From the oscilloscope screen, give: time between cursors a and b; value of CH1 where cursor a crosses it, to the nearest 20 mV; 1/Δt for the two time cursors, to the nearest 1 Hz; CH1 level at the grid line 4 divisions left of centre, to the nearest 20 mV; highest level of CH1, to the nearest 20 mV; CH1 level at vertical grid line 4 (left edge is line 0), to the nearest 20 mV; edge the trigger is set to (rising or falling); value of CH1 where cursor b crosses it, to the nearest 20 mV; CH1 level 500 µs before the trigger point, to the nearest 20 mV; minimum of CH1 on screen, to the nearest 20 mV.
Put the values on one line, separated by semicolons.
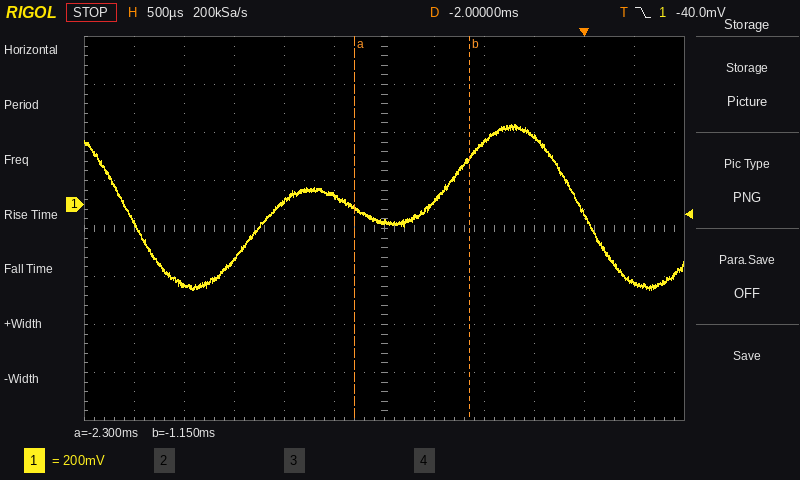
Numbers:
1.15 ms; -20 mV; 870 Hz; -340 mV; 340 mV; 20 mV; falling; 200 mV; 280 mV; -360 mV
